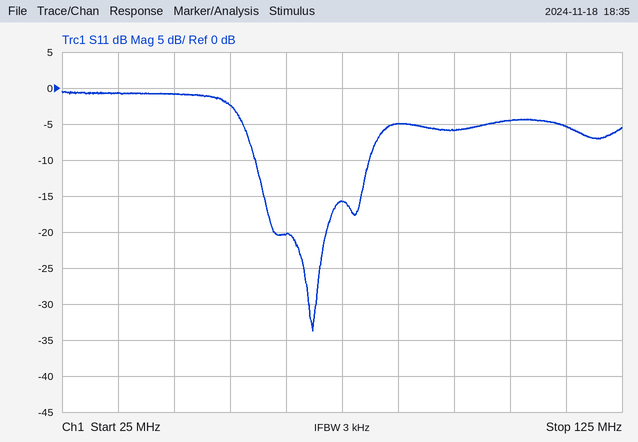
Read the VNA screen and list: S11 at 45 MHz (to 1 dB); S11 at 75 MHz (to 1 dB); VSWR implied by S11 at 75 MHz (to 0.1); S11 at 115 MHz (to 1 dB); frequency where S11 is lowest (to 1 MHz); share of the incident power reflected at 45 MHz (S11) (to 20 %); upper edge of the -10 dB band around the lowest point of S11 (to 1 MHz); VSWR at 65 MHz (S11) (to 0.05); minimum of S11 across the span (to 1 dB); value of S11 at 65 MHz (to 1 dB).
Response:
-1 dB
-16 dB
1.4
-5 dB
70 MHz
80 %
80 MHz
1.20
-34 dB
-20 dB
